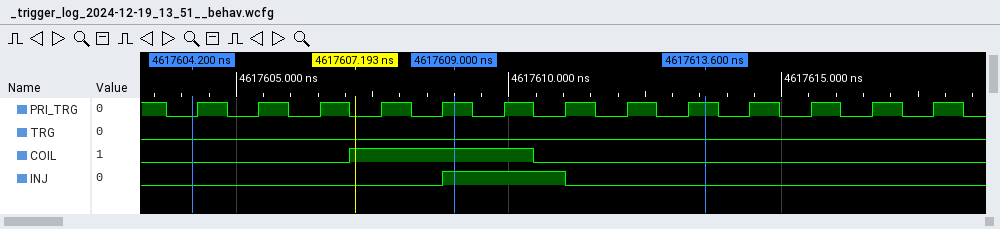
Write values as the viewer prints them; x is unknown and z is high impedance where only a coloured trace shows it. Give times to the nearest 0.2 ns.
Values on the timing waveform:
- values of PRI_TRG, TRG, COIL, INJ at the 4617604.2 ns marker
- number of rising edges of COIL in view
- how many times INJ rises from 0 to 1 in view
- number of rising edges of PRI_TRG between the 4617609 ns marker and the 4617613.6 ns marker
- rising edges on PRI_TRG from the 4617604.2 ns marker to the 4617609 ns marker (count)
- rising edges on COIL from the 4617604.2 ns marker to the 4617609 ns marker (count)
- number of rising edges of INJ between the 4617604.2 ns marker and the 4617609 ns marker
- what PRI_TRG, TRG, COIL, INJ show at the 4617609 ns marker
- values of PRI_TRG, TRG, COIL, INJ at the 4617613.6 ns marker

PRI_TRG=0, TRG=0, COIL=0, INJ=0
1
1
4
5
1
1
PRI_TRG=1, TRG=0, COIL=1, INJ=1
PRI_TRG=1, TRG=0, COIL=0, INJ=0
